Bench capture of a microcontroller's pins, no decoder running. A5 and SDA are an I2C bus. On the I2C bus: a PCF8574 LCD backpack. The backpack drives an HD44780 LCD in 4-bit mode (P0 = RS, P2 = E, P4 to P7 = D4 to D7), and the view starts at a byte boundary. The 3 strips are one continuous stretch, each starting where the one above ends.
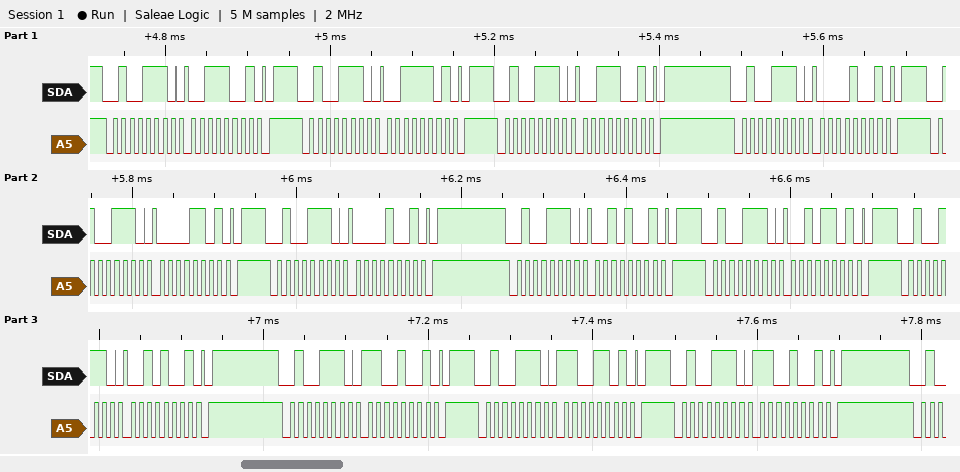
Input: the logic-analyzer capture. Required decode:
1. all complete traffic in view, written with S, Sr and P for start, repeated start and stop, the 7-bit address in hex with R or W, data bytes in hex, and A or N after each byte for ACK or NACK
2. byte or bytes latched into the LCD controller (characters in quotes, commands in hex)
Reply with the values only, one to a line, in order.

S 27W A 39 A P S 27W A 3D A P S 27W A 39 A P S 27W A 09 A P S 27W A 0D A P S 27W A 09 A P S 27W A 29 A P S 27W A 2D A P S 27W A 29 A P S 27W A C9 A P S 27W A CD A P S 27W A C9 A P
'0' ','
